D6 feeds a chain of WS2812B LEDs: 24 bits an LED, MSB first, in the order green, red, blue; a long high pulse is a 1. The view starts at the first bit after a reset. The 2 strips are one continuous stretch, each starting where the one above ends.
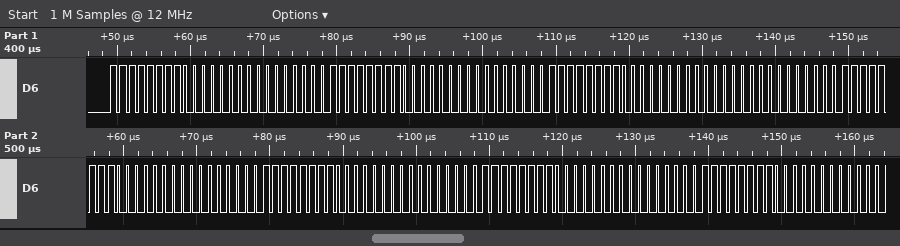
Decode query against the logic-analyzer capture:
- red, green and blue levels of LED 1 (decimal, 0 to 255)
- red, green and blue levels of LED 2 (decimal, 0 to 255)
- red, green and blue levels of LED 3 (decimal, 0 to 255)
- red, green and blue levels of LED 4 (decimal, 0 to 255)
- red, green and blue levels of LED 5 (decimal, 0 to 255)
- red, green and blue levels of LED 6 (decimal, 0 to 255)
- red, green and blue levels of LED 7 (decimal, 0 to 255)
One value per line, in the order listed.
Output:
0, 255, 0
0, 255, 0
0, 255, 0
255, 0, 0
255, 0, 0
255, 0, 0
255, 0, 0
